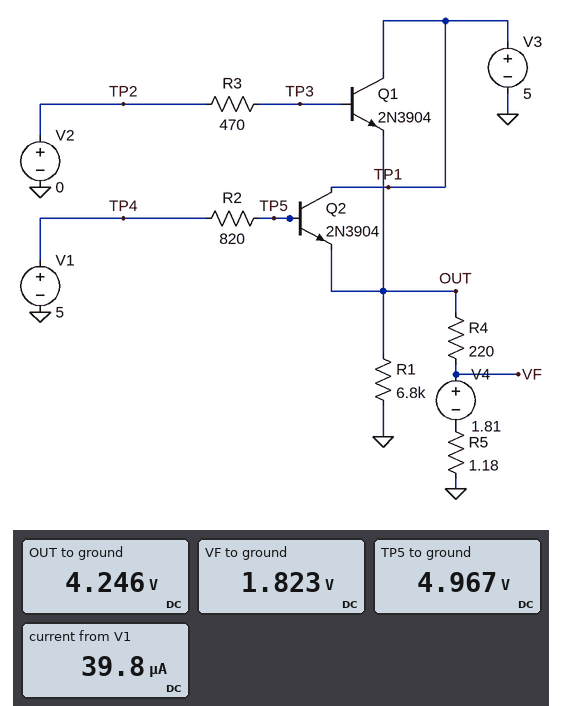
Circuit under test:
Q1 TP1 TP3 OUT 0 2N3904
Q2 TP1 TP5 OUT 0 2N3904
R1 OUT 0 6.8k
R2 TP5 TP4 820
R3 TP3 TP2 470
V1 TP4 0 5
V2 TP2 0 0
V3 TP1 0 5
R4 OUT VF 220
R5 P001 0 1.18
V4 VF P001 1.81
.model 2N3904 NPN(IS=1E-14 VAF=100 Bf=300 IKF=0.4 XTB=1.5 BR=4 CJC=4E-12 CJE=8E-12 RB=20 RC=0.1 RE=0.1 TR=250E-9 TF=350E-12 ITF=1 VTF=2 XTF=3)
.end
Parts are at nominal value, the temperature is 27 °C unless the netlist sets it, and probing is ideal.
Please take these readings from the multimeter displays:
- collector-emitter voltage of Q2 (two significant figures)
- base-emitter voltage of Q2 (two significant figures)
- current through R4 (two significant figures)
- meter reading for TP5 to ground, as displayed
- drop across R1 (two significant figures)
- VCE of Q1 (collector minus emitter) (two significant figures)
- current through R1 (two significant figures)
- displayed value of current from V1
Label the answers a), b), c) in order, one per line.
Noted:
a) 750 mV
b) 720 mV
c) 11 mA
d) 4.967 V
e) 4.2 V
f) 750 mV
g) 620 µA
h) 39.8 µA
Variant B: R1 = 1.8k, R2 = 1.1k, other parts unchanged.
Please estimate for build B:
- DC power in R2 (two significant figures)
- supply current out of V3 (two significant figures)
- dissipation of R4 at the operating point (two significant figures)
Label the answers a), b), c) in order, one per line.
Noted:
a) 2.3 µW
b) 13 mA
c) 26 mW
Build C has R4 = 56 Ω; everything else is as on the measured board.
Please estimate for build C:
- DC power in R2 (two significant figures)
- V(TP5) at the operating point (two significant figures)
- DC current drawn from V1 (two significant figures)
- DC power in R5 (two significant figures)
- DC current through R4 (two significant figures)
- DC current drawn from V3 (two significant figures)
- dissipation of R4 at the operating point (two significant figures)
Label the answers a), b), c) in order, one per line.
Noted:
a) 18 µW
b) 4.9 V
c) 150 µA
d) 1.9 mW
e) 40 mA
f) 41 mA
g) 91 mW
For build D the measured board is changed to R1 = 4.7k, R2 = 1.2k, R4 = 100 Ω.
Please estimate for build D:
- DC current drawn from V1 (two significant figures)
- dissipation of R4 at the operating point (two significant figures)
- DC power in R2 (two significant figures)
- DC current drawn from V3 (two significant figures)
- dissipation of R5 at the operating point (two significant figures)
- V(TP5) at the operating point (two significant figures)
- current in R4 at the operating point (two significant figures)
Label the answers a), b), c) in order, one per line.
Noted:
a) 85 µA
b) 54 mW
c) 8.6 µW
d) 24 mA
e) 630 µW
f) 4.9 V
g) 23 mA
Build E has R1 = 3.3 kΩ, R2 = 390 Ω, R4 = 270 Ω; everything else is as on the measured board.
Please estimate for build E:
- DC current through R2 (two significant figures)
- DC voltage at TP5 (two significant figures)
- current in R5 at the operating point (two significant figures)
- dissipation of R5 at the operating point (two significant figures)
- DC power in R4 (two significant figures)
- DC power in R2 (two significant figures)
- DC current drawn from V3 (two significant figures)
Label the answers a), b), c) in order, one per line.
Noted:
a) 35 µA
b) 5.0 V
c) 9.1 mA
d) 97 µW
e) 22 mW
f) 490 nW
g) 10 mA
